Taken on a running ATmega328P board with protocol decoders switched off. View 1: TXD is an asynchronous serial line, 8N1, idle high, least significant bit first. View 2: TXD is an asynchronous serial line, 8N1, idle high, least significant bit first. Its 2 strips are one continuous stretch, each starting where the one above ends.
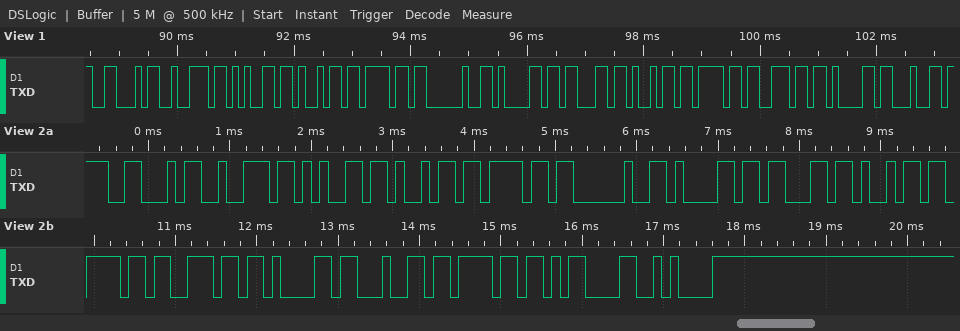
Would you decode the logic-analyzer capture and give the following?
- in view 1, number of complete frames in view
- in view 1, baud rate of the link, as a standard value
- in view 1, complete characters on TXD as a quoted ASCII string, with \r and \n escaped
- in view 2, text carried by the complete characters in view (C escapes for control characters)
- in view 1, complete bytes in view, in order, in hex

13
9600 baud
"Freio acionad"
"Freio acionado\r\n"
46 72 65 69 6F 20 61 63 69 6F 6E 61 64
